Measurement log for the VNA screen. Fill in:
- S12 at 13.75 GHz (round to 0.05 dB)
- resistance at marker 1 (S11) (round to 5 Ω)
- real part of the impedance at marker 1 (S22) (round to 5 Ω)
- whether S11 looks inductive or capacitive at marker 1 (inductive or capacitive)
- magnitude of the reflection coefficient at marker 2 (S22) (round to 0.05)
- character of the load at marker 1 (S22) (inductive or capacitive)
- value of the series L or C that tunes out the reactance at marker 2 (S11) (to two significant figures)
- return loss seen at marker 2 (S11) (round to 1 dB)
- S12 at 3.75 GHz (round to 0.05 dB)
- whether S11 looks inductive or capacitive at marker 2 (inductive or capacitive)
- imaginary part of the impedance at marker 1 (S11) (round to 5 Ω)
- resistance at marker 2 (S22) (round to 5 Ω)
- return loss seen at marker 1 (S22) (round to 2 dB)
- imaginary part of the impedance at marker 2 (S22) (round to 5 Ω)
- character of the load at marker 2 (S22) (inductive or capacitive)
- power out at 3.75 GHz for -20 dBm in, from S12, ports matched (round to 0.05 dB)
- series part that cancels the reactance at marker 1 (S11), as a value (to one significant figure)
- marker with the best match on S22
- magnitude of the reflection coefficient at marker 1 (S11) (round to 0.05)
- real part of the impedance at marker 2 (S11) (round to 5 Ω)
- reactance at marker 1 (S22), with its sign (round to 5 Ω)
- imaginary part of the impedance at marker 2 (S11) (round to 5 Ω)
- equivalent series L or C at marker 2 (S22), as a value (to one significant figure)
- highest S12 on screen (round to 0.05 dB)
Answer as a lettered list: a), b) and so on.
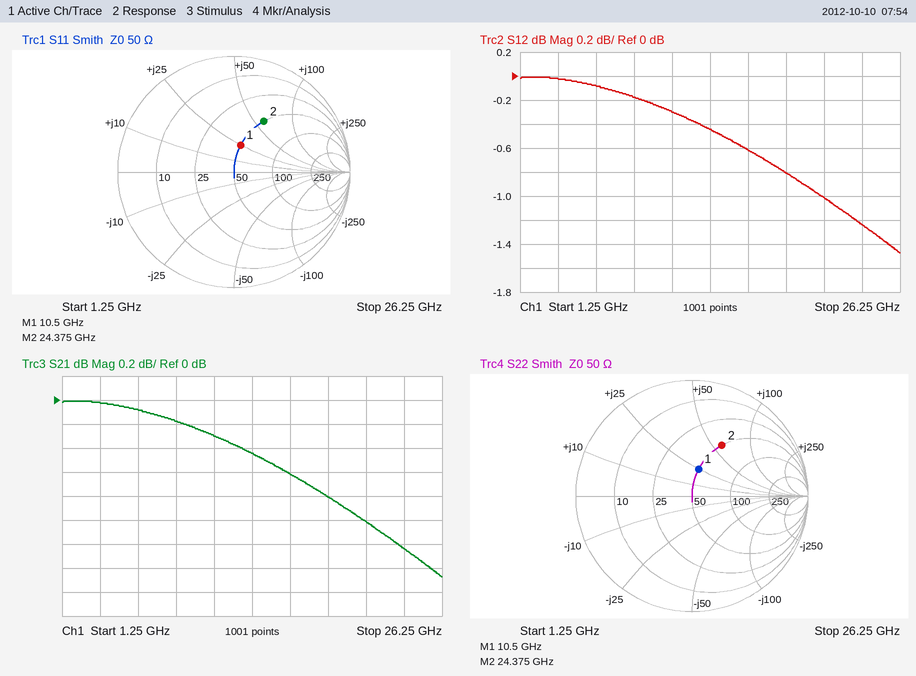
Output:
a) -0.45 dB
b) 50 Ω
c) 50 Ω
d) inductive
e) 0.50
f) inductive
g) 110 fF
h) 6 dB
i) 0.00 dB
j) inductive
k) +25 Ω
l) 50 Ω
m) 12 dB
n) +60 Ω
o) inductive
p) -20.00 dBm
q) 600 fF
r) marker 1
s) 0.25
t) 50 Ω
u) +25 Ω
v) +60 Ω
w) 400 pH
x) 0.00 dB
